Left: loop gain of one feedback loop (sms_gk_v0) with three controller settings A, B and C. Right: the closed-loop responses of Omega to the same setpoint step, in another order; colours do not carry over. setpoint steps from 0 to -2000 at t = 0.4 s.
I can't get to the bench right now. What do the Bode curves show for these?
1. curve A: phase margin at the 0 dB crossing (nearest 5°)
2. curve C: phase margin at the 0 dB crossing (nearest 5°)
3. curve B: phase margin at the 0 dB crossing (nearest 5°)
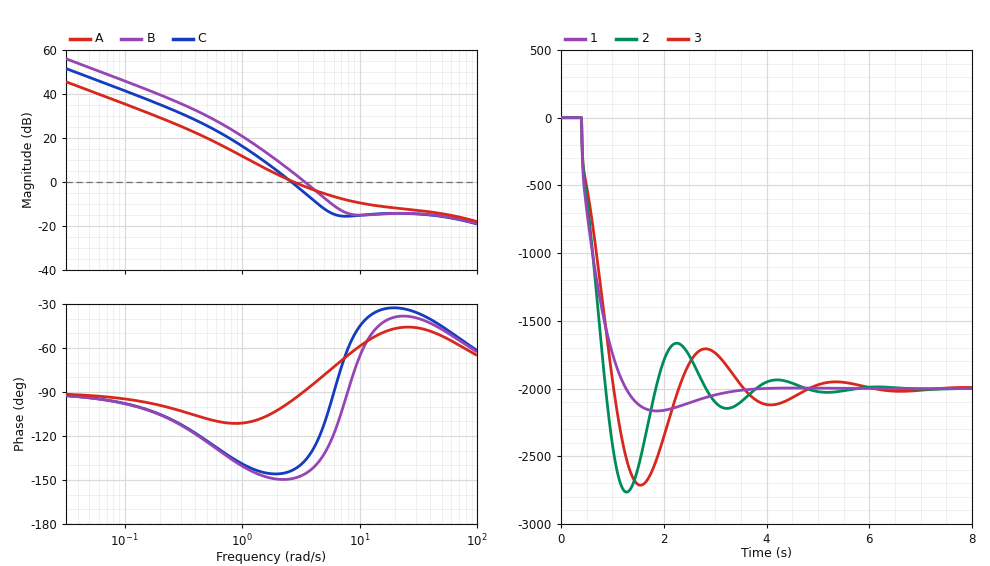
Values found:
85°
35°
35°
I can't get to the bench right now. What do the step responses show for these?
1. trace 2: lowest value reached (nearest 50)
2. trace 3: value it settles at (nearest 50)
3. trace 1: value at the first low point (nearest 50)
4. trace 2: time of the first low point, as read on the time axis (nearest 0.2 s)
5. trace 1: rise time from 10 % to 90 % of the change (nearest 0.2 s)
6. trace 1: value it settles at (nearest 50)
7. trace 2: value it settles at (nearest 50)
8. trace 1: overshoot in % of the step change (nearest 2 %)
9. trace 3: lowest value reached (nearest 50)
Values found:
-2750
-2000
-2150
1.2 s
0.6 s
-2000
-2000
8 %
-2700
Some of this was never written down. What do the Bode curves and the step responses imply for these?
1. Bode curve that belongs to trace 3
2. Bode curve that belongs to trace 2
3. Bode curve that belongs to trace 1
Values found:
C
B
A
